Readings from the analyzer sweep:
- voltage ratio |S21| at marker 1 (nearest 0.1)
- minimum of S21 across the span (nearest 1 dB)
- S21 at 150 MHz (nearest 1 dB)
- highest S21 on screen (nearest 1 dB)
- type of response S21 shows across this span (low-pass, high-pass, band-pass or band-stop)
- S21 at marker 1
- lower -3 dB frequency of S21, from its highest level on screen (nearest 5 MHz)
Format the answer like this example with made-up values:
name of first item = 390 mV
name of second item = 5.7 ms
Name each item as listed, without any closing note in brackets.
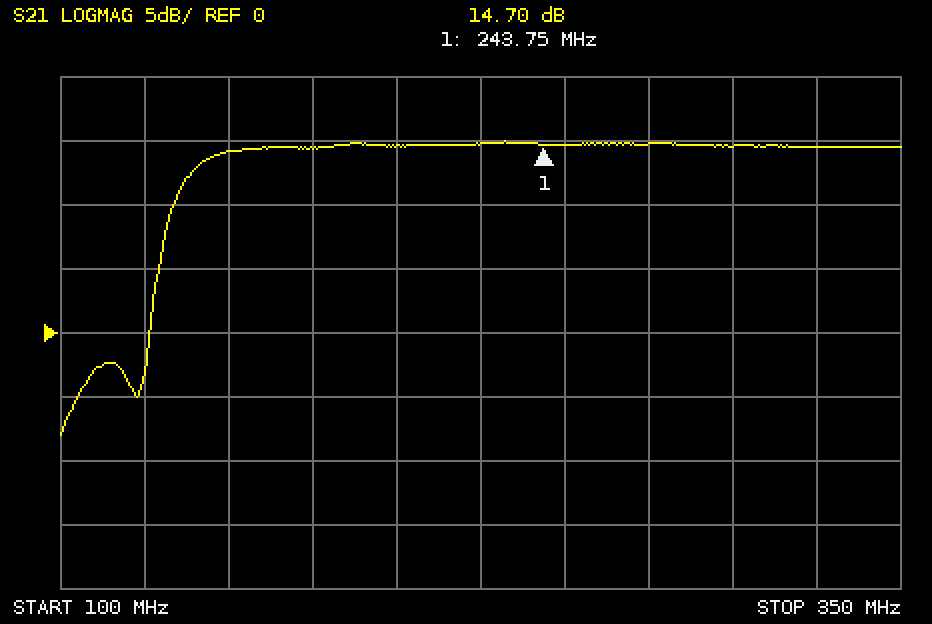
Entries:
voltage ratio |S21| at marker 1 = 5.4
minimum of S21 across the span = -8 dB
S21 at 150 MHz = 14 dB
highest S21 on screen = 15 dB
type of response S21 shows across this span = high-pass
S21 at marker 1 = 14.70 dB
lower -3 dB frequency of S21, from its highest level on screen = 135 MHz
